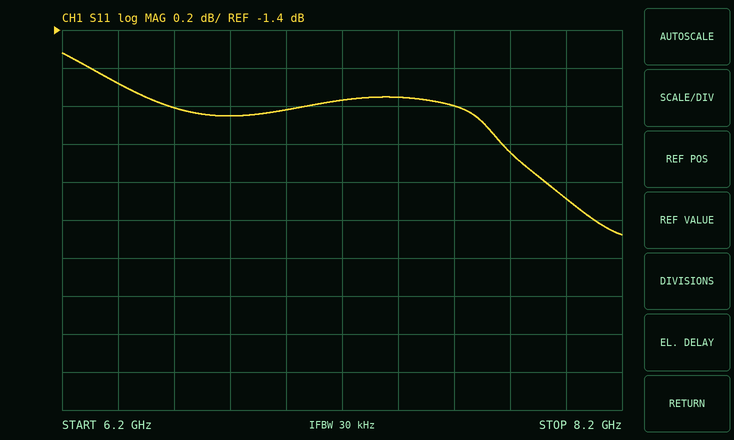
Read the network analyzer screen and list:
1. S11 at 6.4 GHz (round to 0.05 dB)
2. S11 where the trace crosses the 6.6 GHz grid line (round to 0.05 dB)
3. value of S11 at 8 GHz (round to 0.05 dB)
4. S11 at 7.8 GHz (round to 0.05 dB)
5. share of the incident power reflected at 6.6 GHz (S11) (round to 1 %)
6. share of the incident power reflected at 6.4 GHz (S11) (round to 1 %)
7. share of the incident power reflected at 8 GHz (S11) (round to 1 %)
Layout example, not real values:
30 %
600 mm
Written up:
-1.70 dB
-1.80 dB
-2.30 dB
-2.05 dB
66 %
68 %
59 %
